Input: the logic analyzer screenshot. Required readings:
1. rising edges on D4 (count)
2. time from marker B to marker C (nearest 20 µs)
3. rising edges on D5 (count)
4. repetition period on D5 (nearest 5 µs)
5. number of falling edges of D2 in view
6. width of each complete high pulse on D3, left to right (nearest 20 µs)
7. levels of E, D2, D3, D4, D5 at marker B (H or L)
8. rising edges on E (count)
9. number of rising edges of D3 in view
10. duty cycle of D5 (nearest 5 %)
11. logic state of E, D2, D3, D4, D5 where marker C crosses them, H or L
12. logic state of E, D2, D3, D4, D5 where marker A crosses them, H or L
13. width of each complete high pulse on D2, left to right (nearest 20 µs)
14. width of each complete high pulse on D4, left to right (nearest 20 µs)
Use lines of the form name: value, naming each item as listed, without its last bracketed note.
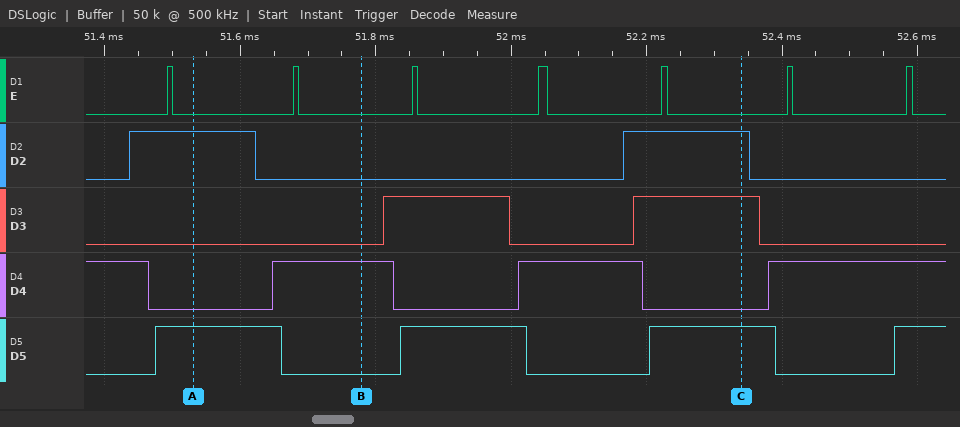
rising edges on D4: 3
time from marker B to marker C: 560 µs
rising edges on D5: 4
repetition period on D5: 365 µs
number of falling edges of D2 in view: 2
width of each complete high pulse on D3, left to right: 180 µs, 180 µs
levels of E, D2, D3, D4, D5 at marker B: E=L, D2=L, D3=L, D4=H, D5=L
rising edges on E: 7
number of rising edges of D3 in view: 2
duty cycle of D5: 50 %
logic state of E, D2, D3, D4, D5 where marker C crosses them, H or L: E=L, D2=H, D3=H, D4=L, D5=H
logic state of E, D2, D3, D4, D5 where marker A crosses them, H or L: E=L, D2=H, D3=L, D4=L, D5=H
width of each complete high pulse on D2, left to right: 180 µs, 180 µs
width of each complete high pulse on D4, left to right: 180 µs, 180 µs
